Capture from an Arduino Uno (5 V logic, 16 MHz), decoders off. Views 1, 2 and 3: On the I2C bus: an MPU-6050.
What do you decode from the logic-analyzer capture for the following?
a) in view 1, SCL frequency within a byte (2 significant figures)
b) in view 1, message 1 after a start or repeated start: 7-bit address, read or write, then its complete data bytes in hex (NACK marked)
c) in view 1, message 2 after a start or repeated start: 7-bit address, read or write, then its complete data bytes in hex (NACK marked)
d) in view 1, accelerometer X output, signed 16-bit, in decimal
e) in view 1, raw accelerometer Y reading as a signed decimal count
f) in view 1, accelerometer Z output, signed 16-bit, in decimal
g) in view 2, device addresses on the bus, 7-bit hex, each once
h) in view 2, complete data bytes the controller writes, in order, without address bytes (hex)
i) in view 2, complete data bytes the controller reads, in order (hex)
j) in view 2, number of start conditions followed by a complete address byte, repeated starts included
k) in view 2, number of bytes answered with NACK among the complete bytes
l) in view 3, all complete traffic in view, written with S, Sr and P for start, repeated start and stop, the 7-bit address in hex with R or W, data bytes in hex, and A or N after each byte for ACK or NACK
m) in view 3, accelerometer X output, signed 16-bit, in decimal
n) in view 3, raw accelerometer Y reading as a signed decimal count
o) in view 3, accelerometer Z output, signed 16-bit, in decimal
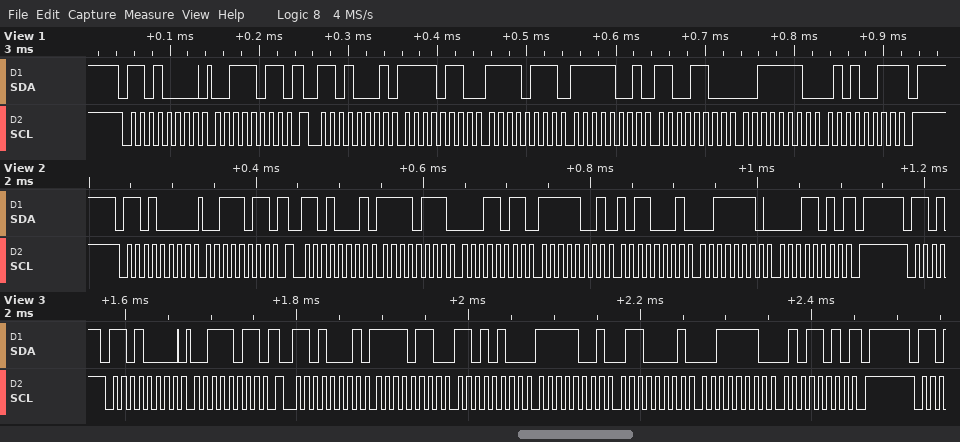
100 kHz
0x68 write: 3B
0x68 read: F6 F7 F9 CC 3E 53 NACK
-2313
-1588
15955
0x68
3B
F7 1B F9 B1 3E 1A
2
1
S 68W A 3B A Sr 68R A F6 A D4 A F9 A 61 A 3E A 5A N P
-2348
-1695
15962
